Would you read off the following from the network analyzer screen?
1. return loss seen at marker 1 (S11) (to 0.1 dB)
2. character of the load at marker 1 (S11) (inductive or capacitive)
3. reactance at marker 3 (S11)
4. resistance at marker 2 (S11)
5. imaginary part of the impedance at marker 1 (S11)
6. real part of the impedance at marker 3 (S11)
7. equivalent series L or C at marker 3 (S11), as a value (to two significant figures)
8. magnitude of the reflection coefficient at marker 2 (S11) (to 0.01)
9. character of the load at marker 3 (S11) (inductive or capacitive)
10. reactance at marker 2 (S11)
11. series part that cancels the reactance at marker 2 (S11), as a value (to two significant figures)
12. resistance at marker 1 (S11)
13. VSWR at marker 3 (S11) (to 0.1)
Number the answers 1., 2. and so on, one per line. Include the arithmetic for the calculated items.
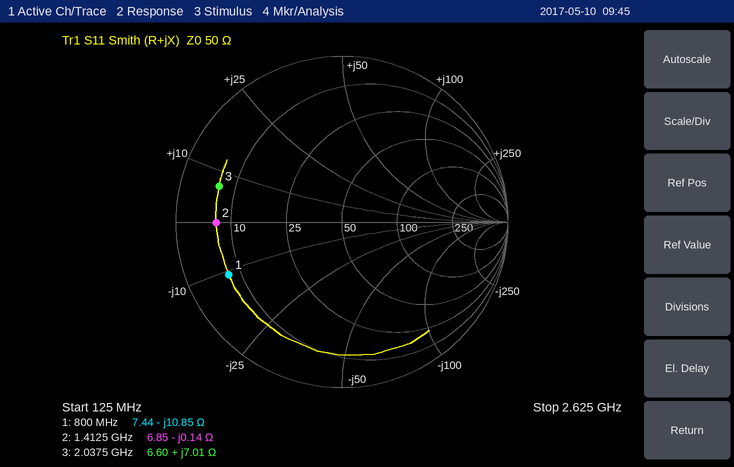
1. 2.5 dB
2. capacitive
3. +7.01 Ω
4. 6.85 Ω
5. -10.85 Ω
6. 6.60 Ω
7. L = 7.01 Ω/(2π × 2.0375 GHz) ≈ 548 pH, so 550 pH to two significant figures
8. 0.76
9. inductive
10. -0.14 Ω
11. L = 0.14 Ω/(2π × 1.4125 GHz) ≈ 16 pH
12. 7.44 Ω
13. 7.7
